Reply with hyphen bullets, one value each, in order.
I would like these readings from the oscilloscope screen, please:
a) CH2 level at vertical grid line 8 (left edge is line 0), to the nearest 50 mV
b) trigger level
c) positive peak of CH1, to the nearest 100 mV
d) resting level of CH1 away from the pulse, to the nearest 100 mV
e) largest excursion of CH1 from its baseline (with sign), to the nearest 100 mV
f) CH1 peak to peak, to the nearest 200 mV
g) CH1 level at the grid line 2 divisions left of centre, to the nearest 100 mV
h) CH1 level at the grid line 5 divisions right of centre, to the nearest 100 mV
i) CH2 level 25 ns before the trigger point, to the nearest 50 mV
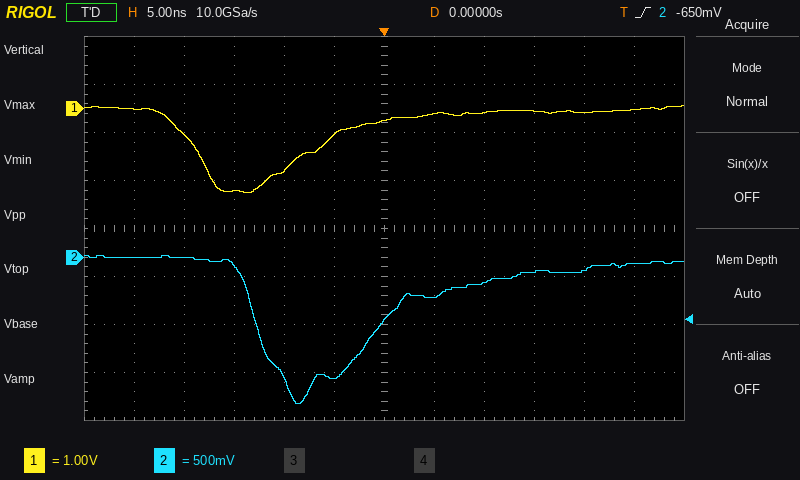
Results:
- -250 mV
- -650 mV
- 100 mV
- -100 mV
- -1.7 V
- 1.8 V
- -1.3 V
- 0.0 V
- 0 mV
